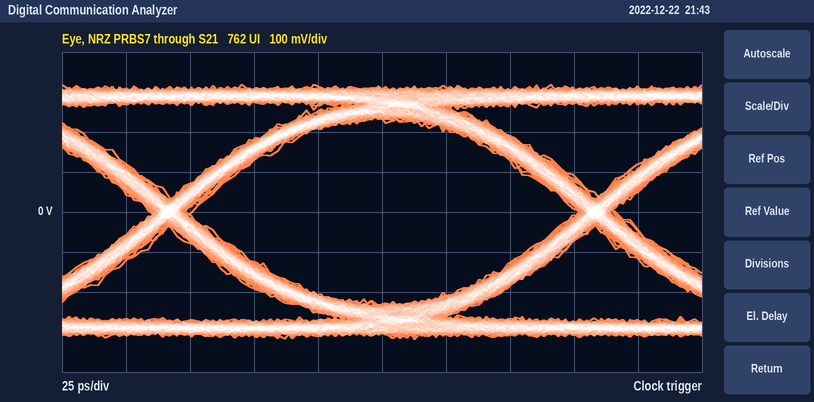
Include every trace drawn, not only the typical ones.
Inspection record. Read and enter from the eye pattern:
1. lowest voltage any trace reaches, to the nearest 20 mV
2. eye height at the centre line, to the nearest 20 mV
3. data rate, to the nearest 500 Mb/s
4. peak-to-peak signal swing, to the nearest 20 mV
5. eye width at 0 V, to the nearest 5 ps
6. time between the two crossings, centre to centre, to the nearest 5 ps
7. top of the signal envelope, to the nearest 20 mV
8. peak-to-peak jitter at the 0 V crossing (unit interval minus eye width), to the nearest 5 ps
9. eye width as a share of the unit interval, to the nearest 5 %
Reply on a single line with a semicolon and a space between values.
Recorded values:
-320 mV; 460 mV; 6.0 Gb/s; 640 mV; 150 ps; 165 ps; 320 mV; 15 ps; 90 %
